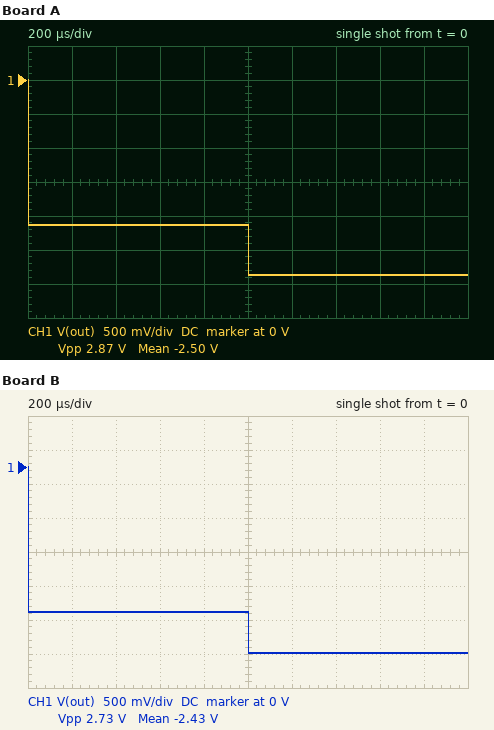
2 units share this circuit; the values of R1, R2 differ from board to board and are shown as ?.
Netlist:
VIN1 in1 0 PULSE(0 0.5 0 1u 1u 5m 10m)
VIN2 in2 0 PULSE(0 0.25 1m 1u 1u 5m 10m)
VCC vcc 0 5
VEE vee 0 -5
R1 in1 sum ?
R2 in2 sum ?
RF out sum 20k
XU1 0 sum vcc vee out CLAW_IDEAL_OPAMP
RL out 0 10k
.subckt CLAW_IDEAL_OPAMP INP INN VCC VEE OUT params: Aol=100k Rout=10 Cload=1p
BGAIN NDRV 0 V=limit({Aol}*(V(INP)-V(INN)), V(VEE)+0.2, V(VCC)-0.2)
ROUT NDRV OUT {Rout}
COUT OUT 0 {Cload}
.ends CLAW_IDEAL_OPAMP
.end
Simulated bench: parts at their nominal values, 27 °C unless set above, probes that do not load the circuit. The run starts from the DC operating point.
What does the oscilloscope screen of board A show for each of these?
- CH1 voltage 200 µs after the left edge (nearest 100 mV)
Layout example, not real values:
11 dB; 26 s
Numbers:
-2.1 V
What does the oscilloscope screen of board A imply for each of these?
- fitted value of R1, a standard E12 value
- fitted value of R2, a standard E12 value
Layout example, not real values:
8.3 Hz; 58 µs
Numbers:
4.7 kΩ; 6.8 kΩ
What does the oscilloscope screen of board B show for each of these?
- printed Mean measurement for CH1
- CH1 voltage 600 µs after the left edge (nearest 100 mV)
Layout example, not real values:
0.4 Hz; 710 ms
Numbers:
-2.43 V; -2.1 V
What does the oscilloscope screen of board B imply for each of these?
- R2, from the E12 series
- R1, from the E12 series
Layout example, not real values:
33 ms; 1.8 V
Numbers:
8.2 kΩ; 4.7 kΩ
